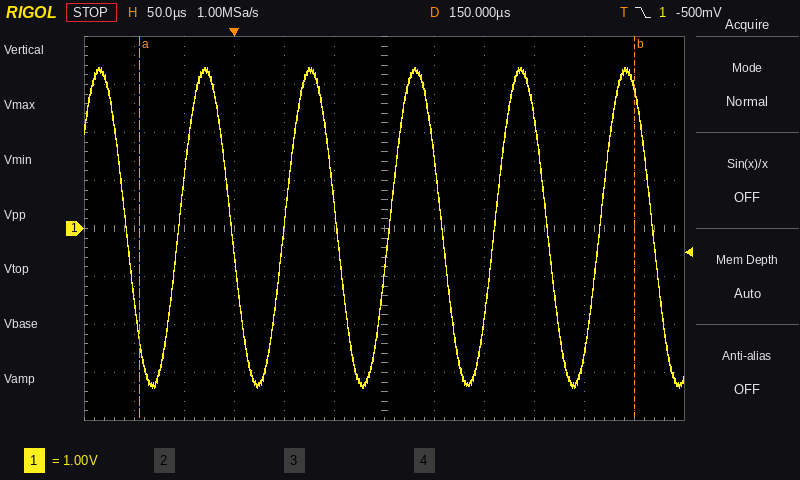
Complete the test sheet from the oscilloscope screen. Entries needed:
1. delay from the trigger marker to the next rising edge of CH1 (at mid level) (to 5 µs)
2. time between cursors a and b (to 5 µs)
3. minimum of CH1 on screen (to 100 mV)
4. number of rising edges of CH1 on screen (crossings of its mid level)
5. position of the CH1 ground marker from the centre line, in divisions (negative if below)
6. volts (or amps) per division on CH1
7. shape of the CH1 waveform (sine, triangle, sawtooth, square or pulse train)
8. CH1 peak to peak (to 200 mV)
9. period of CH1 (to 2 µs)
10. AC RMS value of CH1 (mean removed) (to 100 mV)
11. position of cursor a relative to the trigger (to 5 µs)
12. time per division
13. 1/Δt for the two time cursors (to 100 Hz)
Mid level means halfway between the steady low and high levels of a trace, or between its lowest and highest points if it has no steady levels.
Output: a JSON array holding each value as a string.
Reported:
["50 µs", "495 µs", "-3.3 V", "5", "0.0 div", "1 V", "sine", "6.6 V", "106 µs", "2.3 V", "-95 µs", "50 µs", "2.0 kHz"]
